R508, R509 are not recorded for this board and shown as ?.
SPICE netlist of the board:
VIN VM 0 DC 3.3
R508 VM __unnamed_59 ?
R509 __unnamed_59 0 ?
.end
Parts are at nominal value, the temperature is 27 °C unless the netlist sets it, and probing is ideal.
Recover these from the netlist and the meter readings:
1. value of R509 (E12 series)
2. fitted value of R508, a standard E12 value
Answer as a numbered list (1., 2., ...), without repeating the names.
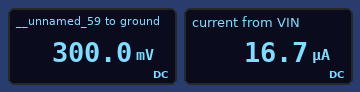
1. 18 kΩ
2. 180 kΩ
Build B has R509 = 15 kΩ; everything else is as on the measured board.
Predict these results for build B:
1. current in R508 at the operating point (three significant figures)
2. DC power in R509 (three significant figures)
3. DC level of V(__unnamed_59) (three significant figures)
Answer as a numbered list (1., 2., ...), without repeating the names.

1. 16.9 µA
2. 4.30 µW
3. 254 mV
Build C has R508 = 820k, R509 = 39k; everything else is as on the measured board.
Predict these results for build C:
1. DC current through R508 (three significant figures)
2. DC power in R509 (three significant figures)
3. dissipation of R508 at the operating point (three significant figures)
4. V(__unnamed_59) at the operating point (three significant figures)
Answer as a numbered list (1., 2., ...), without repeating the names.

1. 3.84 µA
2. 576 nW
3. 12.1 µW
4. 150 mV
